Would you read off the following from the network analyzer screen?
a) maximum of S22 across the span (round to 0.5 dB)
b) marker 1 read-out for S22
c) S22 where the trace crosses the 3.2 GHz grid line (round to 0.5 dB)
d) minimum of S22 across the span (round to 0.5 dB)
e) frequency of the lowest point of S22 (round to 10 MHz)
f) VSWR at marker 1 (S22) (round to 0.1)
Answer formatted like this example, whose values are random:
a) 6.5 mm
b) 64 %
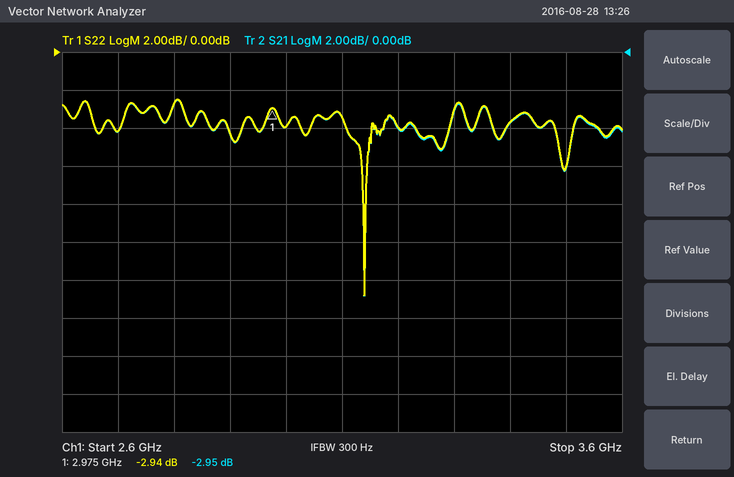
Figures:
a) -2.5 dB
b) -2.94 dB
c) -4.0 dB
d) -13.0 dB
e) 3.14 GHz
f) 6.0
